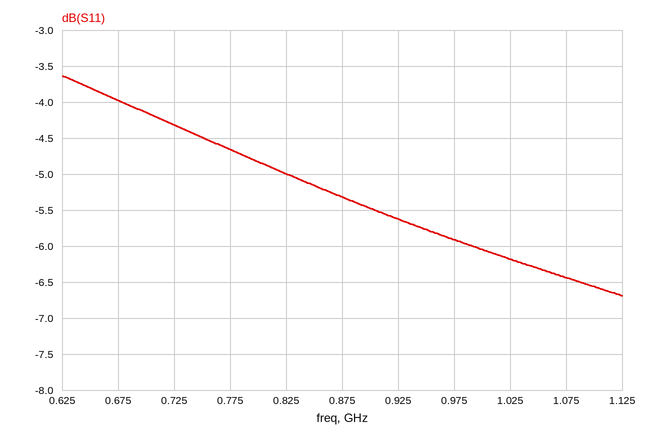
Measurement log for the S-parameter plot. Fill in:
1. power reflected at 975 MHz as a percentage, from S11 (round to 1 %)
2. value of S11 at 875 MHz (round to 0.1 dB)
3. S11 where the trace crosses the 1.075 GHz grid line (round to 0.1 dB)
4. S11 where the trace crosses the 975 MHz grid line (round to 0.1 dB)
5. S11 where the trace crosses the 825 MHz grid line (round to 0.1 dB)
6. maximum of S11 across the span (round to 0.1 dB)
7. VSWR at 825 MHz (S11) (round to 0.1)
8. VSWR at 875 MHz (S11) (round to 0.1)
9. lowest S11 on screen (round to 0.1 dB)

26 %
-5.3 dB
-6.4 dB
-5.9 dB
-5.0 dB
-3.6 dB
3.6
3.4
-6.7 dB
